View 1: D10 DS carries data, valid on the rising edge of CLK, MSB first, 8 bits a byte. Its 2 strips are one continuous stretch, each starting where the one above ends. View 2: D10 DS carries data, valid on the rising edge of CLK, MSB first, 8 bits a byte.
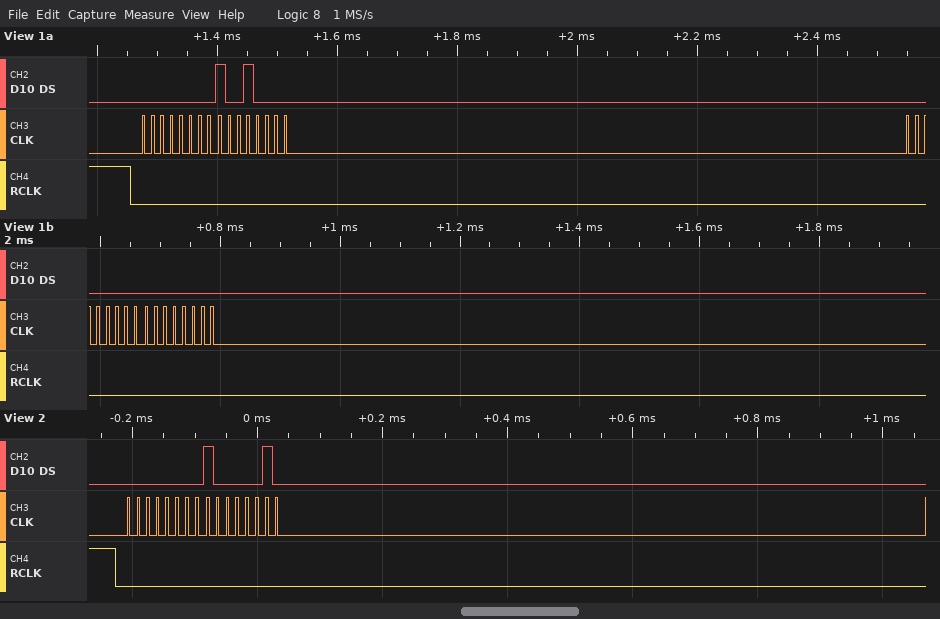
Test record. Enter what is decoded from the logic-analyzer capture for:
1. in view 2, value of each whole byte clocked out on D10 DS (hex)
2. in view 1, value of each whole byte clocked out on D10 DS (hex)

0x00 0x82
00 90 00 00
